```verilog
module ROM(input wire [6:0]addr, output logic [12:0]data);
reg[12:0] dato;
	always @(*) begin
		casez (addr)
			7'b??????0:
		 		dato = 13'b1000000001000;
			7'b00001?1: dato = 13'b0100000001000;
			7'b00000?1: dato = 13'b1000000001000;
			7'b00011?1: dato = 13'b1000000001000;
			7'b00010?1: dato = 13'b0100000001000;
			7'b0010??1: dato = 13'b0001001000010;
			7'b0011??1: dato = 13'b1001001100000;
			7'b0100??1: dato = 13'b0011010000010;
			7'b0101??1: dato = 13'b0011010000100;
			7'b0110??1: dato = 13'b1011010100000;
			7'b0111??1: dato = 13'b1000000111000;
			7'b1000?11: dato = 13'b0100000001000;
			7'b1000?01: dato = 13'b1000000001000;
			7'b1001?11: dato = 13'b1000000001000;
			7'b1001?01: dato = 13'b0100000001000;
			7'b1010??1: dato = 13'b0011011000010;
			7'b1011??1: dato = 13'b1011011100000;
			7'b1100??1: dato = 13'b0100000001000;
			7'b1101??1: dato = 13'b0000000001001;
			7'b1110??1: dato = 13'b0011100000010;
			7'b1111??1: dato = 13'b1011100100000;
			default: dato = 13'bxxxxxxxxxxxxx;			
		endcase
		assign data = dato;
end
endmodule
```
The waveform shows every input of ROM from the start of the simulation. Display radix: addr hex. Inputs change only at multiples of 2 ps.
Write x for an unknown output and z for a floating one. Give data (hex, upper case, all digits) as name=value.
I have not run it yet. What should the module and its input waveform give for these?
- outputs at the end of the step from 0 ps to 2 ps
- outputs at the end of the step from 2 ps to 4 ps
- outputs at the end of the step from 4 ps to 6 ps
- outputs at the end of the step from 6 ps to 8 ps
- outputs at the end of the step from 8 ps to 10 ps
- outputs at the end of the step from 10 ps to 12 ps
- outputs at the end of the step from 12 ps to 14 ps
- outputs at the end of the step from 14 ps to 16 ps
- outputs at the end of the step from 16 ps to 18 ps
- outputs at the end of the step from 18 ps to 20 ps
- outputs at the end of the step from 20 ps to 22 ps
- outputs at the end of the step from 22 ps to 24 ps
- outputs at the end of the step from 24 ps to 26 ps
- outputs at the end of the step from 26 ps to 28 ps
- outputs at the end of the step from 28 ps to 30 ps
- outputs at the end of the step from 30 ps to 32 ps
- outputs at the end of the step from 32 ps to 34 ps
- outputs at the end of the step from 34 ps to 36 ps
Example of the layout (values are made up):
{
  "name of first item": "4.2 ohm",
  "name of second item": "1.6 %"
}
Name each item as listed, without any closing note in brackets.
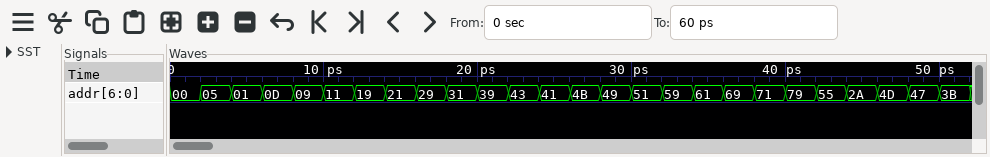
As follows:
{
  "outputs at the end of the step from 0 ps to 2 ps": "data=1008",
  "outputs at the end of the step from 2 ps to 4 ps": "data=0808",
  "outputs at the end of the step from 4 ps to 6 ps": "data=1008",
  "outputs at the end of the step from 6 ps to 8 ps": "data=1008",
  "outputs at the end of the step from 8 ps to 10 ps": "data=0808",
  "outputs at the end of the step from 10 ps to 12 ps": "data=0242",
  "outputs at the end of the step from 12 ps to 14 ps": "data=1260",
  "outputs at the end of the step from 14 ps to 16 ps": "data=0682",
  "outputs at the end of the step from 16 ps to 18 ps": "data=0684",
  "outputs at the end of the step from 18 ps to 20 ps": "data=16A0",
  "outputs at the end of the step from 20 ps to 22 ps": "data=1038",
  "outputs at the end of the step from 22 ps to 24 ps": "data=0808",
  "outputs at the end of the step from 24 ps to 26 ps": "data=1008",
  "outputs at the end of the step from 26 ps to 28 ps": "data=1008",
  "outputs at the end of the step from 28 ps to 30 ps": "data=0808",
  "outputs at the end of the step from 30 ps to 32 ps": "data=06C2",
  "outputs at the end of the step from 32 ps to 34 ps": "data=16E0",
  "outputs at the end of the step from 34 ps to 36 ps": "data=0808"
}
